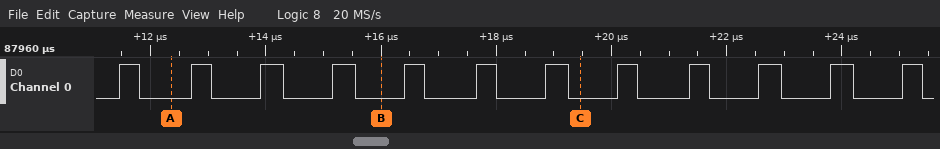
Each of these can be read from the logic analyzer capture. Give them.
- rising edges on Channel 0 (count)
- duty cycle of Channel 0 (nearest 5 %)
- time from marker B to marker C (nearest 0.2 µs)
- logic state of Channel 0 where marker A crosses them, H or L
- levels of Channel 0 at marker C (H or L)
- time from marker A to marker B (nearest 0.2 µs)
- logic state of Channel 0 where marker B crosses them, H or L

12
30 %
3.4 µs
Channel 0=L
Channel 0=L
3.6 µs
Channel 0=L
